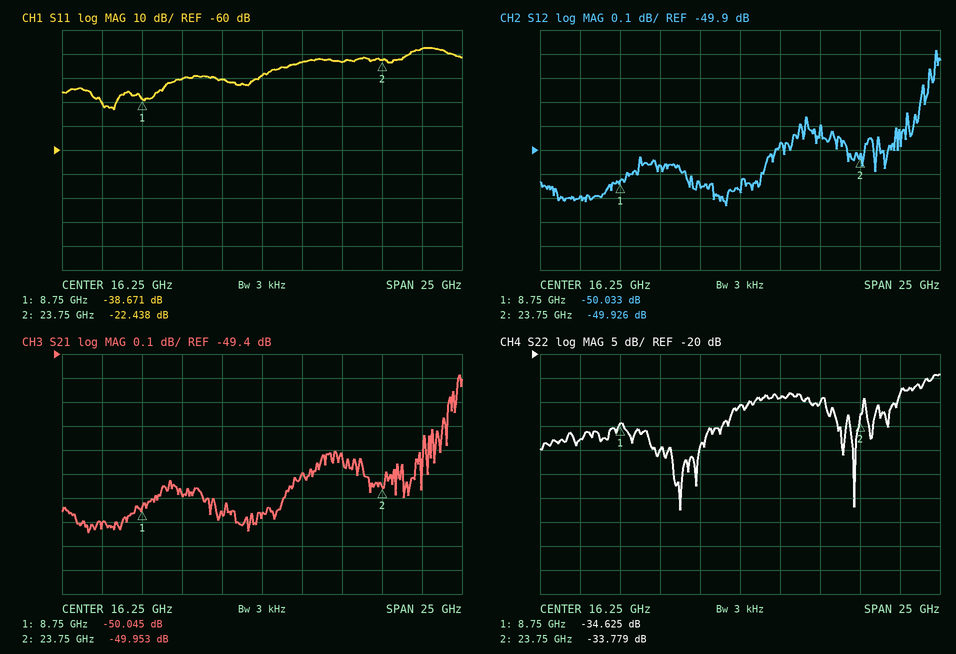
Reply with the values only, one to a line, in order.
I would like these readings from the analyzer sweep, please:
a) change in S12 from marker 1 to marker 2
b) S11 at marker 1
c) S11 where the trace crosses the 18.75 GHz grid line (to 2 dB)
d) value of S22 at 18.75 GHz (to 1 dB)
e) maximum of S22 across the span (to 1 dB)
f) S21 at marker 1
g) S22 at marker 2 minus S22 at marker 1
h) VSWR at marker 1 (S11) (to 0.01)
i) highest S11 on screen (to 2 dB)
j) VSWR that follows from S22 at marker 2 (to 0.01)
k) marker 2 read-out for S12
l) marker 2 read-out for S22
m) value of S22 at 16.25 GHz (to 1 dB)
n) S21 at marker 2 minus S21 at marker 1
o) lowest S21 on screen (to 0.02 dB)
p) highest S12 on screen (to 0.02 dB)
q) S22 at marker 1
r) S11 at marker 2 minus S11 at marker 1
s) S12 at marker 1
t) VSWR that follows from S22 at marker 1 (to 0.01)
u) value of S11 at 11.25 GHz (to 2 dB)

0.107 dB
-38.671 dB
-24 dB
-29 dB
-24 dB
-50.045 dB
0.846 dB
1.02
-18 dB
1.04
-49.926 dB
-33.779 dB
-31 dB
0.092 dB
-50.14 dB
-49.48 dB
-34.625 dB
16.233 dB
-50.033 dB
1.04
-30 dB
